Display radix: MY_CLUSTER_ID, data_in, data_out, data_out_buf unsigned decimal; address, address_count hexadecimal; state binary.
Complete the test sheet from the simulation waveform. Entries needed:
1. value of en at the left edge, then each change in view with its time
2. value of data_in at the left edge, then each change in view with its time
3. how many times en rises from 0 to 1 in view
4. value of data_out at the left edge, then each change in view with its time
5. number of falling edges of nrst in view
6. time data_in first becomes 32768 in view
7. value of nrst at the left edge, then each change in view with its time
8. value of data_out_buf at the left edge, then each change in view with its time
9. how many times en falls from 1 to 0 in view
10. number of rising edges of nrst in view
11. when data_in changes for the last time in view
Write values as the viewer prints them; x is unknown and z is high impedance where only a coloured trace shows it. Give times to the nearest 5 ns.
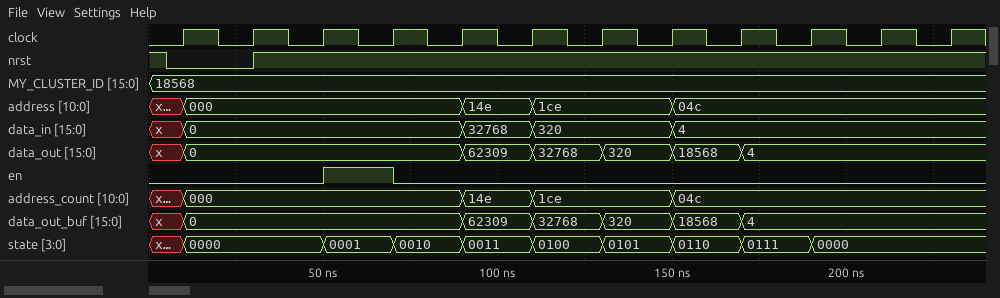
0, 1 at 50 ns, 0 at 70 ns
x, 0 at 10 ns, 32768 at 90 ns, 320 at 110 ns, 4 at 150 ns
1
x, 0 at 10 ns, 62309 at 90 ns, 32768 at 110 ns, 320 at 130 ns, 18568 at 150 ns, 4 at 170 ns
1
90 ns
1, 0 at 5 ns, 1 at 30 ns
x, 0 at 10 ns, 62309 at 90 ns, 32768 at 110 ns, 320 at 130 ns, 18568 at 150 ns, 4 at 170 ns
1
1
150 ns
